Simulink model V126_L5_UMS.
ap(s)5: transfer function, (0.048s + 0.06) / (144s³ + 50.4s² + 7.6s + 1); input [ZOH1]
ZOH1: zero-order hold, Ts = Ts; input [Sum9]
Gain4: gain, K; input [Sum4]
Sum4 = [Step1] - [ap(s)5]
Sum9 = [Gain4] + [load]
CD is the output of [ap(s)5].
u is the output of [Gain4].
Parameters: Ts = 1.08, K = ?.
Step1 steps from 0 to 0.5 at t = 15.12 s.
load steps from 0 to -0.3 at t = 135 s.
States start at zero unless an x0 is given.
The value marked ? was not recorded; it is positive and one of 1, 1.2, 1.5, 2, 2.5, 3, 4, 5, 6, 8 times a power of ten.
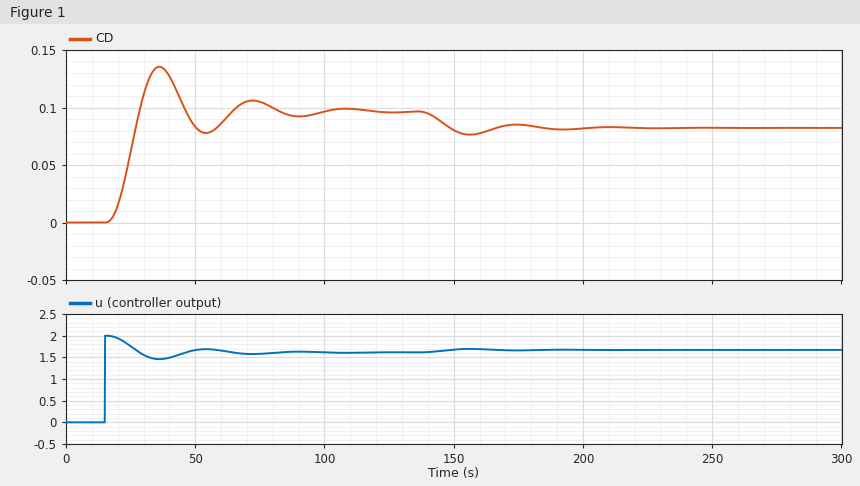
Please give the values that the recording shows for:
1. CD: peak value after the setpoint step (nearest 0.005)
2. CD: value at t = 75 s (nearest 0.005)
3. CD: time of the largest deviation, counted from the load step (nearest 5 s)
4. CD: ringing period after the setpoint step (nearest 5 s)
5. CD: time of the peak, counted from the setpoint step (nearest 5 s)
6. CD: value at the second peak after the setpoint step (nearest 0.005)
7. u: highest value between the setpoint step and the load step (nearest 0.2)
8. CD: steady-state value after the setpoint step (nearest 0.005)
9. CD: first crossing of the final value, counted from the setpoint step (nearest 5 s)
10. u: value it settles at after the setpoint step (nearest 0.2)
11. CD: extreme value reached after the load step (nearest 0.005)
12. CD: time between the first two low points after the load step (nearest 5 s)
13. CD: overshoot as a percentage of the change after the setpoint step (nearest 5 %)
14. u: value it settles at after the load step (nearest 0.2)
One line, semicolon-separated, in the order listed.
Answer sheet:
0.135; 0.105; 20 s; 35 s; 20 s; 0.105; 2.0; 0.095; 15 s; 1.6; 0.075; 35 s; 40 %; 1.6
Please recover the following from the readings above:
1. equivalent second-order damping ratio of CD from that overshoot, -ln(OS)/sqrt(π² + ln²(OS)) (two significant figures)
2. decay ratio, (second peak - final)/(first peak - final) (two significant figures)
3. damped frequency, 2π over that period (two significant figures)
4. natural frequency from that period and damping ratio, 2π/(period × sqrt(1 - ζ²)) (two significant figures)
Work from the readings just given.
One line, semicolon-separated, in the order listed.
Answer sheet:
0.28; 0.25; 0.18 rad/s; 0.19 rad/s
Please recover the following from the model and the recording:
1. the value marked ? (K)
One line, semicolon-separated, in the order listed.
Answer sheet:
4
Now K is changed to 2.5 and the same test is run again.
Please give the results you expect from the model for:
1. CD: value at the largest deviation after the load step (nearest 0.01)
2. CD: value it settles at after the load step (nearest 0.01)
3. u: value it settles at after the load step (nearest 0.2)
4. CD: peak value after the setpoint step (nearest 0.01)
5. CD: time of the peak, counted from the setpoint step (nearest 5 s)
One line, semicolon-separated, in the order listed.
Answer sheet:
0.04; 0.05; 1.2; 0.09; 20 s
